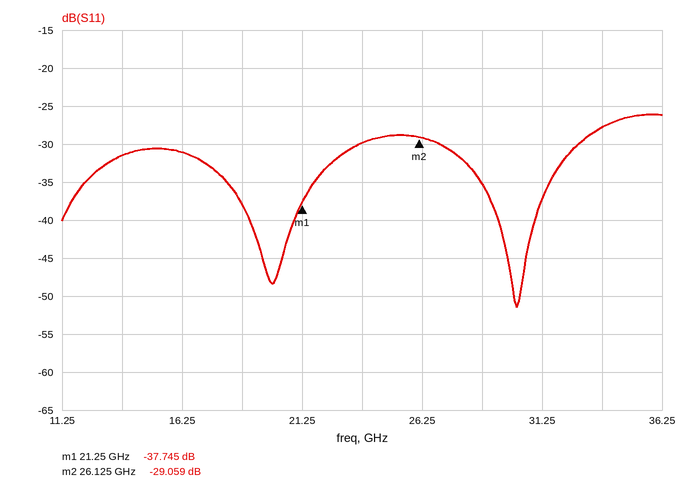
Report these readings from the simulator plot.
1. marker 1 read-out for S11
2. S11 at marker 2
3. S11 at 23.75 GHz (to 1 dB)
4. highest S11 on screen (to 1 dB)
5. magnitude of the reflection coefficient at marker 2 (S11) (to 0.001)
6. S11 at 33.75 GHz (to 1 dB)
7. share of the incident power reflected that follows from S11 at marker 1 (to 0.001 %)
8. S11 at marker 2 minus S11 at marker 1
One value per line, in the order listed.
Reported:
-37.745 dB
-29.059 dB
-30 dB
-26 dB
0.035
-28 dB
0.017 %
8.686 dB
